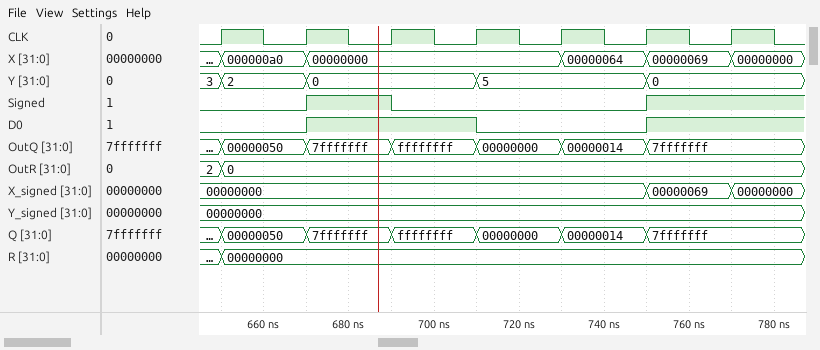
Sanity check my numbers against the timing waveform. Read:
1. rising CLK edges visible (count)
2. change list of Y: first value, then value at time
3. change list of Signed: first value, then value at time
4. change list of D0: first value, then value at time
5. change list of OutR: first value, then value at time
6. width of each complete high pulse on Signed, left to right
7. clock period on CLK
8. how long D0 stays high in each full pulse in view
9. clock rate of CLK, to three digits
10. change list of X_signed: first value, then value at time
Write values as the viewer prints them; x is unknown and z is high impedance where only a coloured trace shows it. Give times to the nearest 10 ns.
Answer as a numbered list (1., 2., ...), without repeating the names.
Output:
1. 7
2. 3, 2 at 650 ns, 0 at 670 ns, 5 at 710 ns, 0 at 750 ns
3. 0, 1 at 670 ns, 0 at 690 ns, 1 at 750 ns
4. 0, 1 at 670 ns, 0 at 710 ns, 1 at 750 ns
5. 2, 0 at 650 ns
6. 20 ns
7. 20 ns
8. 40 ns
9. 50.0 MHz
10. 00000000, 00000069 at 750 ns, 00000000 at 770 ns
